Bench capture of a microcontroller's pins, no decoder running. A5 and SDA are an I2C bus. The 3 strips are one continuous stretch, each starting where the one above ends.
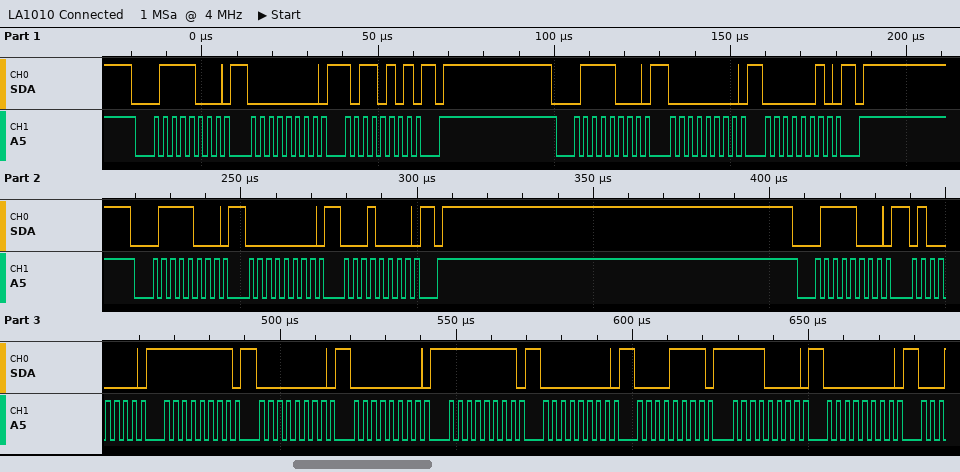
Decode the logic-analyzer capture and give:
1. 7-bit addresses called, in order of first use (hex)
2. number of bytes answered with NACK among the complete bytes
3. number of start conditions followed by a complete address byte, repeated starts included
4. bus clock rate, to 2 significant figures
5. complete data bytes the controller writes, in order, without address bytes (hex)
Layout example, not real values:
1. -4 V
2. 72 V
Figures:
1. 0x3C
2. 0
3. 4
4. 400 kHz
5. 00 B5 00 02 00 10 40 FF 00 00 FF 00 0F F0 00
